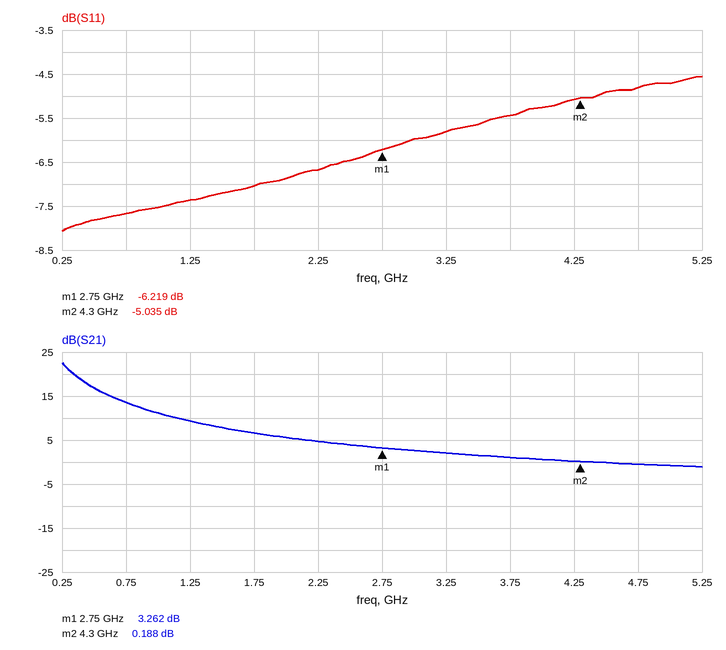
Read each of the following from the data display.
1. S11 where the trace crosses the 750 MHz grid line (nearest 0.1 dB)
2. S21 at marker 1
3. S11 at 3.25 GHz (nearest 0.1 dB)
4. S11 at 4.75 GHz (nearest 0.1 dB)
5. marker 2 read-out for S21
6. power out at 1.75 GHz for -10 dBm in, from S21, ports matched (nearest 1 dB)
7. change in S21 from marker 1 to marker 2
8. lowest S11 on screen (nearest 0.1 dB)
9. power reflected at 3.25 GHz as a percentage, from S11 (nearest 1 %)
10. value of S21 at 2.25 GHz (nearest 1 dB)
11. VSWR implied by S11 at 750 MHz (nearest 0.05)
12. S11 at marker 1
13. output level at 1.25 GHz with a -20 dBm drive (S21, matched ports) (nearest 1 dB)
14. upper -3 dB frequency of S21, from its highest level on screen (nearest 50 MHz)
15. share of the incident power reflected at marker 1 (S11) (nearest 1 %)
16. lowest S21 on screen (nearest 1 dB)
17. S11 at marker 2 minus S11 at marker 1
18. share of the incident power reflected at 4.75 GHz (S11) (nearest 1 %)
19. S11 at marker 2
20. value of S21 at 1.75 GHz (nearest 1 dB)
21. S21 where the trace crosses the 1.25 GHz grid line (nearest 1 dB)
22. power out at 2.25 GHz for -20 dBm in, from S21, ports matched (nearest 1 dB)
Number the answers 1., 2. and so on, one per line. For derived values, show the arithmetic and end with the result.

1. -7.7 dB
2. 3.262 dB
3. -5.8 dB
4. -4.8 dB
5. 0.188 dB
6. -10 dBm + (7 dB) = -3 dBm
7. 0.188 − (3.262) = -3.074 dB
8. -8.1 dB
9. 10^(-5.8/10) ≈ 26 %
10. 5 dB
11. |Γ| = 10^(-7.7/20) = 0.4121; VSWR = (1 + 0.4121)/(1 − 0.4121) ≈ 2.40
12. -6.219 dB
13. -20 dBm + (9 dB) = -11 dBm
14. 350 MHz
15. 10^(-6.219/10) ≈ 24 %
16. -1 dB
17. -5.035 − (-6.219) = 1.184 dB
18. 10^(-4.8/10) ≈ 33 %
19. -5.035 dB
20. 7 dB
21. 9 dB
22. -20 dBm + (5 dB) = -15 dBm
